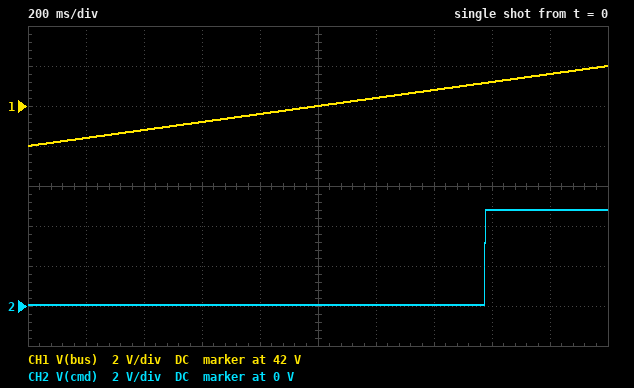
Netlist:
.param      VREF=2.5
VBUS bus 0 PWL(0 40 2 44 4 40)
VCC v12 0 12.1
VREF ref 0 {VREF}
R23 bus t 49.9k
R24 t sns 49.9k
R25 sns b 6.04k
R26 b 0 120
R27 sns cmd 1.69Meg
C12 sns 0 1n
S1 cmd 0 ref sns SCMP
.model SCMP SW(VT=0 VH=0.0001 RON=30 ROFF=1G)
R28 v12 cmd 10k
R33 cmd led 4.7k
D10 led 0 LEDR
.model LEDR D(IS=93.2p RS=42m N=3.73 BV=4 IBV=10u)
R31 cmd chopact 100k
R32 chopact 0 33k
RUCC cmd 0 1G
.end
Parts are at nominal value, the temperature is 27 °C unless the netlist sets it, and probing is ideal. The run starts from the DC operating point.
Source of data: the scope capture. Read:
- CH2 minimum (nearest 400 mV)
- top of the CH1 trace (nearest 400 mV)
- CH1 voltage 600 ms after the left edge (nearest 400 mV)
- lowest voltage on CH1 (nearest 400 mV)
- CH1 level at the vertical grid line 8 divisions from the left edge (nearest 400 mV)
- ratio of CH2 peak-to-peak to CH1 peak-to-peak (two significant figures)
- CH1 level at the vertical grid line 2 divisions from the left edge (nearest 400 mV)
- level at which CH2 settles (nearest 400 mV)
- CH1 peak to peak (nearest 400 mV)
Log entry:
0 V
44.0 V
41.2 V
40.0 V
43.2 V
1.2
40.8 V
4.8 V
4.0 V
